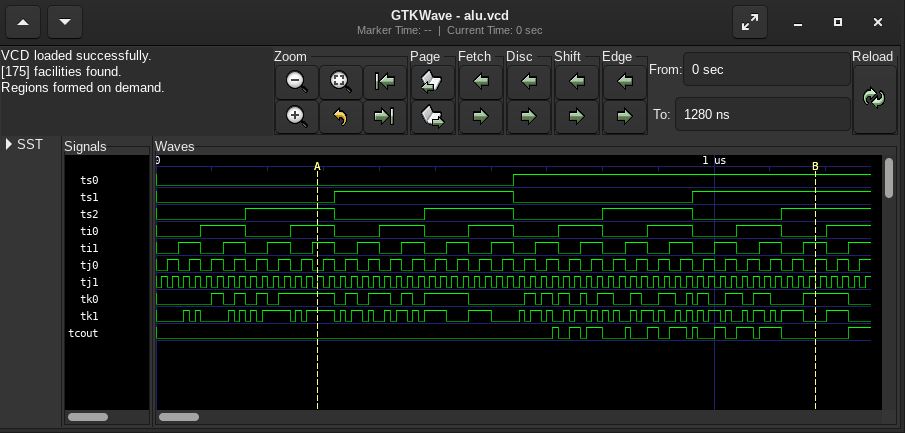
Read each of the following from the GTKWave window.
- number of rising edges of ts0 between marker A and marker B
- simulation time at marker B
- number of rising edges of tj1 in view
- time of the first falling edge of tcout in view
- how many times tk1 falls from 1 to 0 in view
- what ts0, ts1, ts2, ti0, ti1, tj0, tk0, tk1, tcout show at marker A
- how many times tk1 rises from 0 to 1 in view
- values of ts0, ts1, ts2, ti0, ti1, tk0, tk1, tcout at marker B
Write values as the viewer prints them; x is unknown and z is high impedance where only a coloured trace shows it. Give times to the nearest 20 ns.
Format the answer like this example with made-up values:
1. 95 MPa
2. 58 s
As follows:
1. 1
2. 1180 ns
3. 64
4. 720 ns
5. 37
6. ts0=0, ts1=0, ts2=1, ti0=1, ti1=1, tj0=0, tk0=1, tk1=1, tcout=0
7. 37
8. ts0=1, ts1=1, ts2=1, ti0=0, ti1=1, tk0=1, tk1=0, tcout=0
